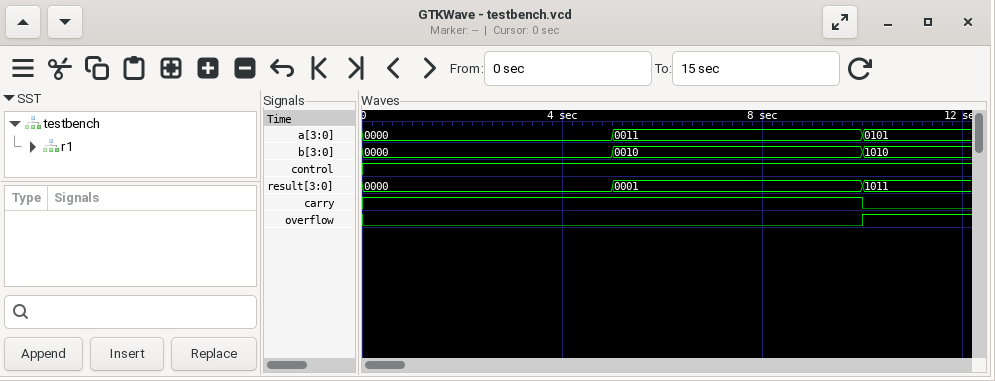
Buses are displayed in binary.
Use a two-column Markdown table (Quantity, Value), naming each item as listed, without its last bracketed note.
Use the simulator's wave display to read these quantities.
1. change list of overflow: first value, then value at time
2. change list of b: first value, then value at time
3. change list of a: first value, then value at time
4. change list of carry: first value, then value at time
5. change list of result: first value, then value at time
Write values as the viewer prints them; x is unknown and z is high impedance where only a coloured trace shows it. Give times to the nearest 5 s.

| Quantity | Value |
|---|---|
| change list of overflow: first value, then value at time | 0, 1 at 10 s |
| change list of b: first value, then value at time | 0000, 0010 at 5 s, 1010 at 10 s |
| change list of a: first value, then value at time | 0000, 0011 at 5 s, 0101 at 10 s |
| change list of carry: first value, then value at time | 1, 0 at 10 s |
| change list of result: first value, then value at time | 0000, 0001 at 5 s, 1011 at 10 s |
